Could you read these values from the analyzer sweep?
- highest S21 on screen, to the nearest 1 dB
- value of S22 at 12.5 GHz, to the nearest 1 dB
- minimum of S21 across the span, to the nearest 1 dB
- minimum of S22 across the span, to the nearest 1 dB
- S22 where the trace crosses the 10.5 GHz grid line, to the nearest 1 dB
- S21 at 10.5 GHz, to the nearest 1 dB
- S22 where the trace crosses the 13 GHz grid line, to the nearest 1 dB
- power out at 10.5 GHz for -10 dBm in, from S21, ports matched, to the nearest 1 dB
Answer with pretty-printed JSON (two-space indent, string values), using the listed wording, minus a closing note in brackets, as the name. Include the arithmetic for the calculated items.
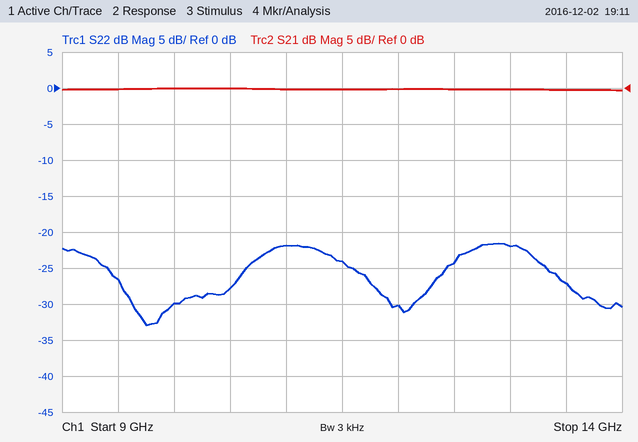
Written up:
{
  "highest S21 on screen, to the nearest 1 dB": "0 dB",
  "value of S22 at 12.5 GHz, to the nearest 1 dB": "-24 dB",
  "minimum of S21 across the span, to the nearest 1 dB": "0 dB",
  "minimum of S22 across the span, to the nearest 1 dB": "-33 dB",
  "S22 where the trace crosses the 10.5 GHz grid line, to the nearest 1 dB": "-28 dB",
  "S21 at 10.5 GHz, to the nearest 1 dB": "0 dB",
  "S22 where the trace crosses the 13 GHz grid line, to the nearest 1 dB": "-22 dB",
  "power out at 10.5 GHz for -10 dBm in, from S21, ports matched, to the nearest 1 dB": "-10 dBm + (0 dB) = -10 dBm"
}
